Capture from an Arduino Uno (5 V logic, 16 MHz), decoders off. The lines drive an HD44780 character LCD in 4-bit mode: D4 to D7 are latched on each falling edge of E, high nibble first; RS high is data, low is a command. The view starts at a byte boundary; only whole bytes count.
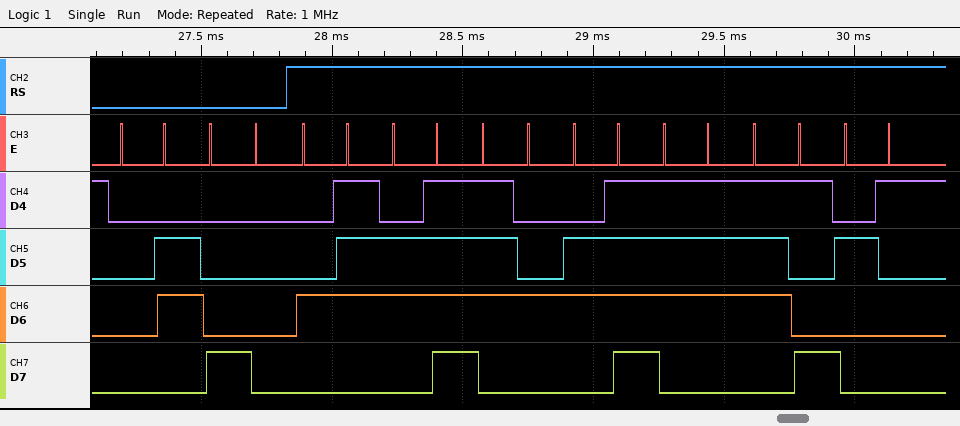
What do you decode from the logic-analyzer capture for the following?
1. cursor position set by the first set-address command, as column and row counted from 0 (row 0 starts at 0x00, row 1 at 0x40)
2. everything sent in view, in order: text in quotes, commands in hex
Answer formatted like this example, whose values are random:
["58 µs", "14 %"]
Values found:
["column 0, row 0", "0x06 0x80 \"Gotowy!\""]
